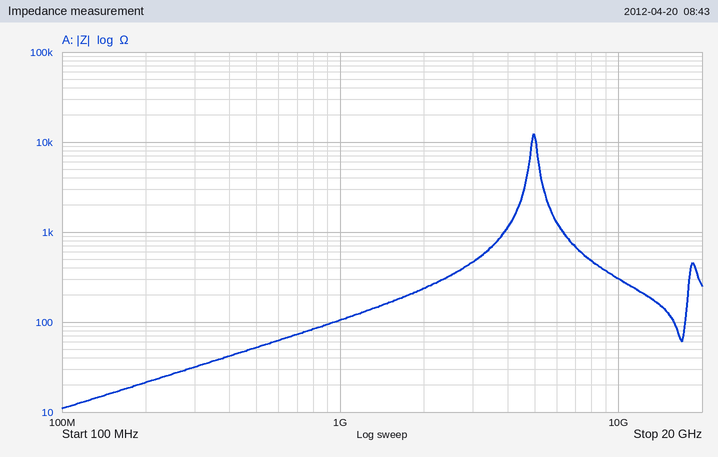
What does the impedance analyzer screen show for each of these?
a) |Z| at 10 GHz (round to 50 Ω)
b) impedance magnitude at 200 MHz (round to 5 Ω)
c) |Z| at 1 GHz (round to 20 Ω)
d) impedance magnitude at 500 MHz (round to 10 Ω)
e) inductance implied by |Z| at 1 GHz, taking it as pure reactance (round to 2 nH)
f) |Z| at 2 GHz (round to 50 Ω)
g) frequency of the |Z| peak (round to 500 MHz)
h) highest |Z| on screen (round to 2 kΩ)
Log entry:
300 Ω
20 Ω
100 Ω
50 Ω
16 nH
250 Ω
5.0 GHz
12 kΩ
